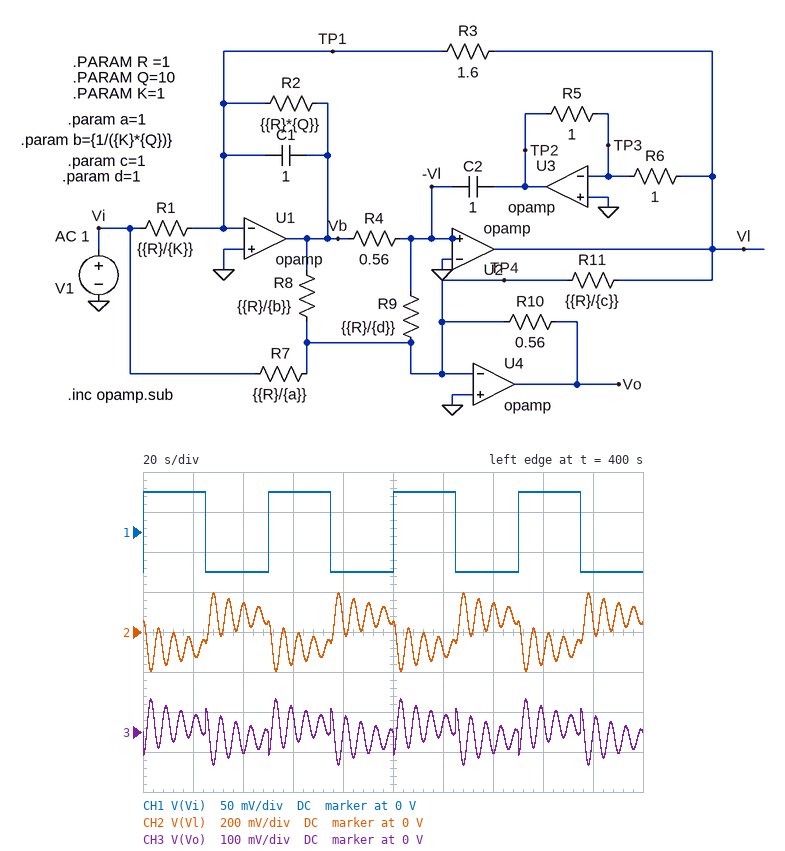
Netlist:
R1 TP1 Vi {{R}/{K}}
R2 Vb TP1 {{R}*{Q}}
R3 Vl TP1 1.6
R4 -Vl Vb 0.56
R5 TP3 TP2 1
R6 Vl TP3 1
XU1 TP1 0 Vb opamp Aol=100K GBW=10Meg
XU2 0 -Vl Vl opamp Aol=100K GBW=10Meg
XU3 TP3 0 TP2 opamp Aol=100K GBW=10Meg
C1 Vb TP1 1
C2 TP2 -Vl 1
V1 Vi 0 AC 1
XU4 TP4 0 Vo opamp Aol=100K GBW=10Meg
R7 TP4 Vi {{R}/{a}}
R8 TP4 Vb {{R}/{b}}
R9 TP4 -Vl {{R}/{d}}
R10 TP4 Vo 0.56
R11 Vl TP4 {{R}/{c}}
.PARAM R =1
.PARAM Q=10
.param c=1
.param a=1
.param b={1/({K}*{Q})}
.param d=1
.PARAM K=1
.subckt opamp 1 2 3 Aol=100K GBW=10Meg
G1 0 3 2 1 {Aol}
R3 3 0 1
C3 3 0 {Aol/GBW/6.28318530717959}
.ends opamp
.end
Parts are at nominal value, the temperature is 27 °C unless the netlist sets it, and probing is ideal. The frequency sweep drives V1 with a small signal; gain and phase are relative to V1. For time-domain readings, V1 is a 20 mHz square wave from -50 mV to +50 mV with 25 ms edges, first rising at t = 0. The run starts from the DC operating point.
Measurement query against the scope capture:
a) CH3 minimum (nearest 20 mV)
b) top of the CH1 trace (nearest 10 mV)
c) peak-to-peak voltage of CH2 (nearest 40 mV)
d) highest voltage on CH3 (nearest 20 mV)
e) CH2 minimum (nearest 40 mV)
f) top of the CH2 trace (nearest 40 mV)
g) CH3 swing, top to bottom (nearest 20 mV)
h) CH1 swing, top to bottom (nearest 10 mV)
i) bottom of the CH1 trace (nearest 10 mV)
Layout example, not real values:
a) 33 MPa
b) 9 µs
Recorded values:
a) -80 mV
b) 50 mV
c) 400 mV
d) 80 mV
e) -200 mV
f) 200 mV
g) 160 mV
h) 100 mV
i) -50 mV
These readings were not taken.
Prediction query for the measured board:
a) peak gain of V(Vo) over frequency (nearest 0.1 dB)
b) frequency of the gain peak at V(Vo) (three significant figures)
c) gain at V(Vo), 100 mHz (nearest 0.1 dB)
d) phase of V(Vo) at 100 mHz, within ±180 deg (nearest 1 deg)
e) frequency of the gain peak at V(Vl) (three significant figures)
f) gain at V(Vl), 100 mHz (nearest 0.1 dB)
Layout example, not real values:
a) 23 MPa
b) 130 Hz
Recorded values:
a) 19.5 dB
b) 168 mHz
c) -1.7 dB
d) -5 deg
e) 168 mHz
f) 7.8 dB
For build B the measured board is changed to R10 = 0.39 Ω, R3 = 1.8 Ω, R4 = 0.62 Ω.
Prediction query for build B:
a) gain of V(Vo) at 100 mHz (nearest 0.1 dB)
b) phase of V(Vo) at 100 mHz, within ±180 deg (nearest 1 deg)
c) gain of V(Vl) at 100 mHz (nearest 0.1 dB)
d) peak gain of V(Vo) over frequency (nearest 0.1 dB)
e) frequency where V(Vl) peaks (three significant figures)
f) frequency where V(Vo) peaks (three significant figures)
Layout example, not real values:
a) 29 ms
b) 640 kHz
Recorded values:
a) -1.3 dB
b) -7 deg
c) 10.1 dB
d) 16.4 dB
e) 150 mHz
f) 151 mHz
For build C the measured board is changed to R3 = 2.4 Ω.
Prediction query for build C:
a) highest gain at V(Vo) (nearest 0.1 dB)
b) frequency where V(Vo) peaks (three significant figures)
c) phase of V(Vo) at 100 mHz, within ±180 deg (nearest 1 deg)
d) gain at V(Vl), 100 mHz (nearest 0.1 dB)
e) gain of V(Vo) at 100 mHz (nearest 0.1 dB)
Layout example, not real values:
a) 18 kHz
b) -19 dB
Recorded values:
a) 21.3 dB
b) 137 mHz
c) -10 deg
d) 14.0 dB
e) 7.1 dB
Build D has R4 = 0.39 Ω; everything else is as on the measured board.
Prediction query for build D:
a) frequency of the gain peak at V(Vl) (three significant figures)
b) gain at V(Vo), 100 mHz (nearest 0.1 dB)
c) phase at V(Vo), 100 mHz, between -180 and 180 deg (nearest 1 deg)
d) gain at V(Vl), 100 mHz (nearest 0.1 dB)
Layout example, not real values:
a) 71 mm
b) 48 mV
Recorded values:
a) 201 mHz
b) -4.0 dB
c) -3 deg
d) 6.5 dB
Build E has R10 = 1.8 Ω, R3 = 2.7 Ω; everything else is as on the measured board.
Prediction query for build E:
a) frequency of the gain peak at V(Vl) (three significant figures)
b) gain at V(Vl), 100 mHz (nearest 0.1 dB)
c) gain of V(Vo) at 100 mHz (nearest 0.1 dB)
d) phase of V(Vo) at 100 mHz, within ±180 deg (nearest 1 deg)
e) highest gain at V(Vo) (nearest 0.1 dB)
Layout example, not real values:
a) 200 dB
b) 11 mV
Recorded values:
a) 129 mHz
b) 16.3 dB
c) 20.0 dB
d) -13 deg
e) 31.9 dB
